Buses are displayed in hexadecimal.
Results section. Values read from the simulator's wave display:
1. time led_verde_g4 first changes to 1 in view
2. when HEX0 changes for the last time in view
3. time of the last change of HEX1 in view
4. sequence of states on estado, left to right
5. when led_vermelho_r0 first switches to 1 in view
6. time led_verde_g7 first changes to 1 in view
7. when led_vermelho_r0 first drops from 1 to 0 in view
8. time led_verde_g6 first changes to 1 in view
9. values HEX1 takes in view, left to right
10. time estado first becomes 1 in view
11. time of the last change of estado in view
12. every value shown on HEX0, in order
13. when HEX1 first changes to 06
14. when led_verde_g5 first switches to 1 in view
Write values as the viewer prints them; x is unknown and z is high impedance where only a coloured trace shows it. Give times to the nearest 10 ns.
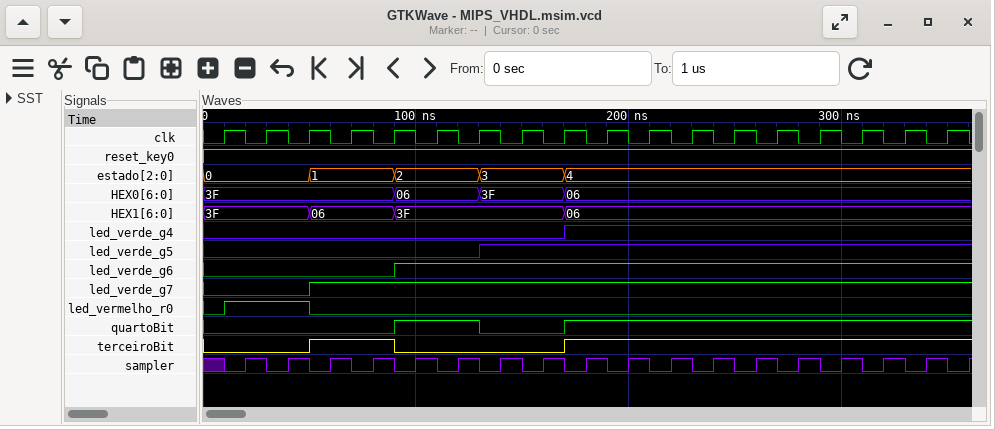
170 ns
170 ns
170 ns
0, 1, 2, 3, 4
10 ns
50 ns
50 ns
90 ns
3F, 06, 3F, 06
50 ns
170 ns
3F, 06, 3F, 06
50 ns
130 ns
